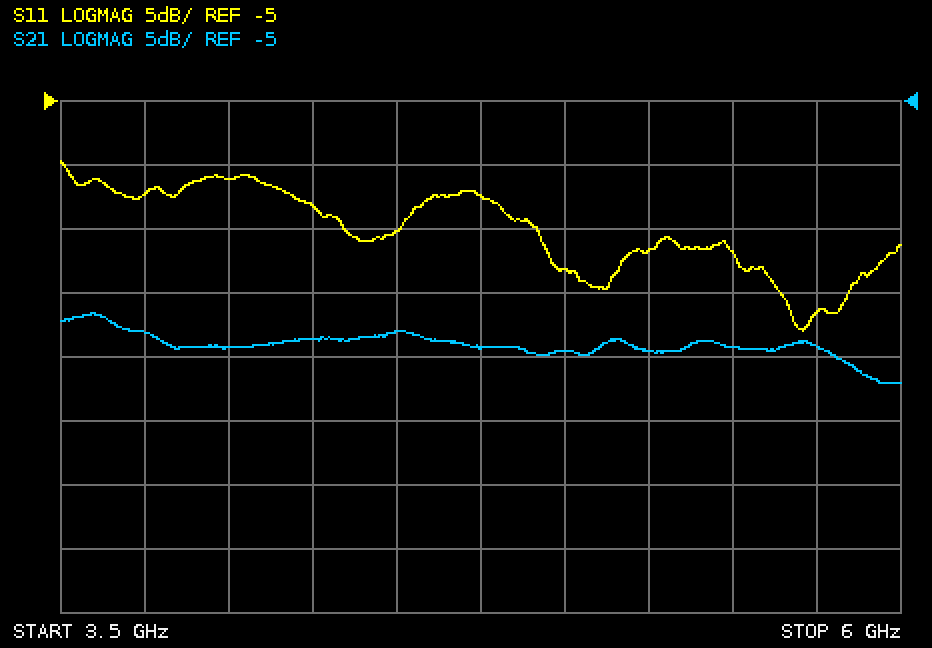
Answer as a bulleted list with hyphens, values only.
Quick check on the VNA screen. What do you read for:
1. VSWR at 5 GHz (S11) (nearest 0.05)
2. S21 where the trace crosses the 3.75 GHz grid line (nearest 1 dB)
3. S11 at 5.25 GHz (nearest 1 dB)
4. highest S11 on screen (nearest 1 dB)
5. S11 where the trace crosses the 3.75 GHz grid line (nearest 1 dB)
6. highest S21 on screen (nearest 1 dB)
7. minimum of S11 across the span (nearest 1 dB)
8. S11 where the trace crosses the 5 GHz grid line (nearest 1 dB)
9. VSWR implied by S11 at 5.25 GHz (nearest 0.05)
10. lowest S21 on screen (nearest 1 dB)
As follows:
- 1.30
- -23 dB
- -17 dB
- -10 dB
- -12 dB
- -22 dB
- -23 dB
- -18 dB
- 1.35
- -27 dB
